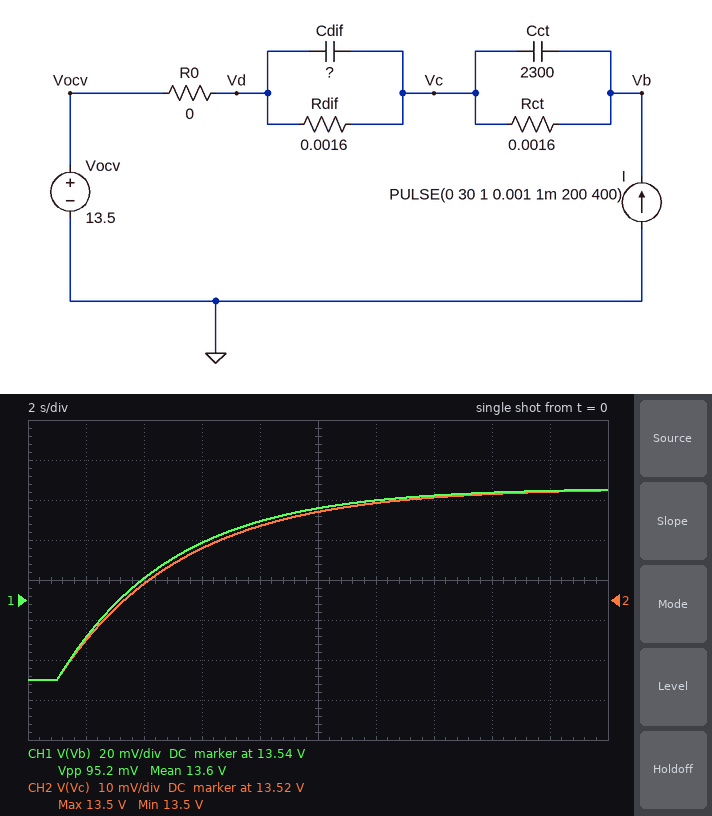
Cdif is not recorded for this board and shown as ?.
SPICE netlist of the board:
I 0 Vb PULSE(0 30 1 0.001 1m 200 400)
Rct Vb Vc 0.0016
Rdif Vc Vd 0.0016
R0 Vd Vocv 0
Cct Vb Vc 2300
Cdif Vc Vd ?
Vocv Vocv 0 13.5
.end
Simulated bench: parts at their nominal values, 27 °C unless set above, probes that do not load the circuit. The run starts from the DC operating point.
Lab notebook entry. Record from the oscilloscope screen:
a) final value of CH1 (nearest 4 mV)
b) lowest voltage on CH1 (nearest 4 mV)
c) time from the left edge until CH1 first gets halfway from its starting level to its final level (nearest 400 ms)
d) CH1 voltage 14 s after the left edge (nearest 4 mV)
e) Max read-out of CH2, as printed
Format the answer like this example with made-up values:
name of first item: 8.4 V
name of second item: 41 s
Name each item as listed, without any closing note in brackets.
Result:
final value of CH1: 13.596 V
lowest voltage on CH1: 13.500 V
time from the left edge until CH1 first gets halfway from its starting level to its final level: 3.6 s
CH1 voltage 14 s after the left edge: 13.592 V
Max read-out of CH2, as printed: 13.5 V
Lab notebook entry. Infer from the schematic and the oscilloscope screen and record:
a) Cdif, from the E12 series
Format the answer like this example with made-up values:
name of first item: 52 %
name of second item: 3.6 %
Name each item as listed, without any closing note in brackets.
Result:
Cdif, from the E12 series: 2.7 kF
